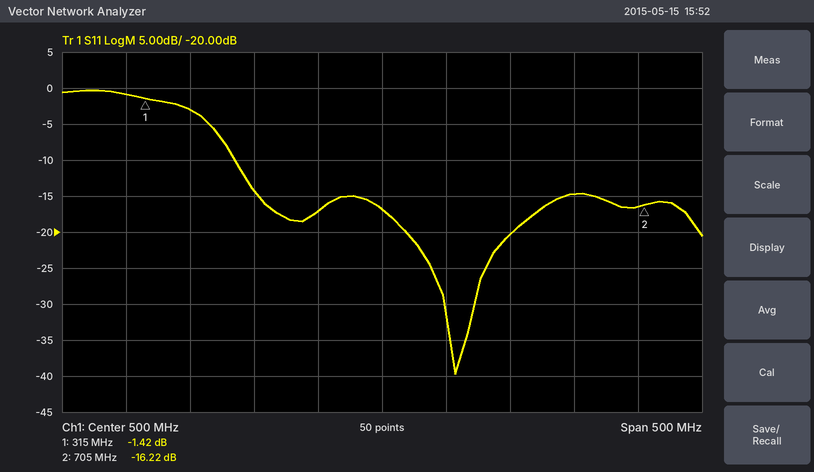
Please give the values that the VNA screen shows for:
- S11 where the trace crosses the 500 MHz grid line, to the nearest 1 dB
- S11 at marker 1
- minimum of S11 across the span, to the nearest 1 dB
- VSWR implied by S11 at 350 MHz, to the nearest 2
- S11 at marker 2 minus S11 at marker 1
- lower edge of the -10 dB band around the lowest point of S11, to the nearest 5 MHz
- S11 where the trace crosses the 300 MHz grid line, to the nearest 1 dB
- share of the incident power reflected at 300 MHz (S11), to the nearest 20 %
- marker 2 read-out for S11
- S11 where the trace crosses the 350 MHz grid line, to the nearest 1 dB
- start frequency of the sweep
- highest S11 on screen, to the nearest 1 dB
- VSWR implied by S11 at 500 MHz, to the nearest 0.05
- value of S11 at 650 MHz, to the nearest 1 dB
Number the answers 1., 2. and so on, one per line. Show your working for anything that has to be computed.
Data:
1. -17 dB
2. -1.42 dB
3. -40 dB
4. |Γ| = 10^(-3/20) = 0.7079; VSWR = (1 + 0.7079)/(1 − 0.7079) ≈ 6
5. -16.22 − (-1.42) = -14.80 dB
6. 385 MHz
7. -1 dB
8. 10^(-1/10) ≈ 79.4 %, so 80 % to the nearest 20 %
9. -16.22 dB
10. -3 dB
11. 250 MHz
12. 0 dB
13. |Γ| = 10^(-17/20) = 0.1413; VSWR = (1 + 0.1413)/(1 − 0.1413) ≈ 1.33, so 1.35 to the nearest 0.05
14. -15 dB
